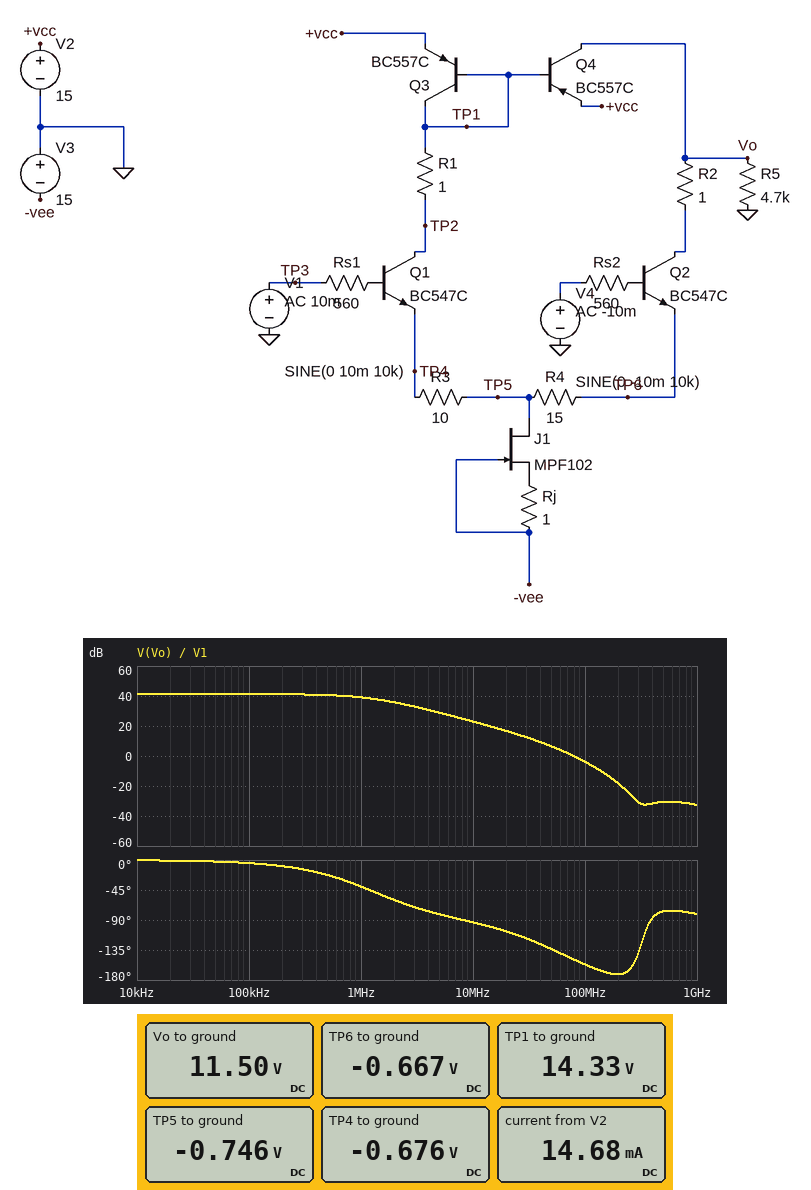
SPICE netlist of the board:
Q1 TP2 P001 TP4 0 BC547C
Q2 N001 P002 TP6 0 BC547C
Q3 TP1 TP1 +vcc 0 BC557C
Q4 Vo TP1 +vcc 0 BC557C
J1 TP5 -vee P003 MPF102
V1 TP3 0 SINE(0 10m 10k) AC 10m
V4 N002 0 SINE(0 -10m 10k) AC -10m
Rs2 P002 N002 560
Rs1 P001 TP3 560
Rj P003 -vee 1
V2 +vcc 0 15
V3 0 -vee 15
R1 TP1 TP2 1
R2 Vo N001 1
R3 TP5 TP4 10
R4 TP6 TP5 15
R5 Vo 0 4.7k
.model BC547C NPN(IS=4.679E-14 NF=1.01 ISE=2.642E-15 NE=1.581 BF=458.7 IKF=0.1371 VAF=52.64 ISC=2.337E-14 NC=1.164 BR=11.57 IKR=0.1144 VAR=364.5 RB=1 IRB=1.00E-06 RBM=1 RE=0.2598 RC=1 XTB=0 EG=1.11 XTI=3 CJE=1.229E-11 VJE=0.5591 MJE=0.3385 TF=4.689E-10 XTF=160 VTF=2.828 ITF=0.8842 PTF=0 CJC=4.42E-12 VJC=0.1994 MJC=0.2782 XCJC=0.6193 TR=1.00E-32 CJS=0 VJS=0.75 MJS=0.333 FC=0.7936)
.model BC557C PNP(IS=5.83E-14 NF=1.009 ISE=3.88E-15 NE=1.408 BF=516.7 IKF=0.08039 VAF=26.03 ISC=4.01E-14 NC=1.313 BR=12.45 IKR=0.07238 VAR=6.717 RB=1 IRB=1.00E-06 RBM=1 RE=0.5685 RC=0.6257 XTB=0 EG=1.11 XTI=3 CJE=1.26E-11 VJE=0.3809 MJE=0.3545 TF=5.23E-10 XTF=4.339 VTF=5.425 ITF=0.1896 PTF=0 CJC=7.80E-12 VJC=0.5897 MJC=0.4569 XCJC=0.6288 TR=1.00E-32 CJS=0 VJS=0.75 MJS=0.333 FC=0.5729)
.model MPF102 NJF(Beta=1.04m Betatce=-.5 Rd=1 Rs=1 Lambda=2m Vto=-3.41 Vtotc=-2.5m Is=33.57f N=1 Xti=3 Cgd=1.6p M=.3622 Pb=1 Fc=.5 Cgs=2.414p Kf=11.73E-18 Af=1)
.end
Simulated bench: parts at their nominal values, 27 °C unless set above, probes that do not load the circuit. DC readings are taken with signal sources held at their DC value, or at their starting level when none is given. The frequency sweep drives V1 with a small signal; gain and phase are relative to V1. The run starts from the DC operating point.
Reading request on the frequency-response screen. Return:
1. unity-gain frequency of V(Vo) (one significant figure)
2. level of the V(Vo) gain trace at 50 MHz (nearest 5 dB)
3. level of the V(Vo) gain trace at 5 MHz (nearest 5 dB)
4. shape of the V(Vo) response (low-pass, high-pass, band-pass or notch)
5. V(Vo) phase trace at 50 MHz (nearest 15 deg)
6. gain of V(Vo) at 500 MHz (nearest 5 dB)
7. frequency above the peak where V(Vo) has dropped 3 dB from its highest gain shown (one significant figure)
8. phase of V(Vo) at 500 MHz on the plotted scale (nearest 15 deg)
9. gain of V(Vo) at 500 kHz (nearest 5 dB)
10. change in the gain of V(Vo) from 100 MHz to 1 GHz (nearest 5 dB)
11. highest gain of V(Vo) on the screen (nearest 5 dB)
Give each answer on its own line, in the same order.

80 MHz
5 dB
30 dB
low-pass
-135 deg
-30 dB
1 MHz
-75 deg
40 dB
-30 dB
40 dB
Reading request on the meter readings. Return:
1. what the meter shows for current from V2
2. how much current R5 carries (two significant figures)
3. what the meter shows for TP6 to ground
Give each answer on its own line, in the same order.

14.68 mA
2.4 mA
-0.667 V
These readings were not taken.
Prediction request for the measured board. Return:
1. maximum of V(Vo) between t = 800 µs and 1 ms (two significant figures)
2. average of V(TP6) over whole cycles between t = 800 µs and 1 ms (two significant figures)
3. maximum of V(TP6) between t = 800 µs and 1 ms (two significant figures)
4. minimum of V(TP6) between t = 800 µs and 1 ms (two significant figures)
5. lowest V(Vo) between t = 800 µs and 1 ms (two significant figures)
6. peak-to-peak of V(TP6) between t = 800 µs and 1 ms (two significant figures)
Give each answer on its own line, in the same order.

14 V
-670 mV
-660 mV
-670 mV
9.1 V
11 mV
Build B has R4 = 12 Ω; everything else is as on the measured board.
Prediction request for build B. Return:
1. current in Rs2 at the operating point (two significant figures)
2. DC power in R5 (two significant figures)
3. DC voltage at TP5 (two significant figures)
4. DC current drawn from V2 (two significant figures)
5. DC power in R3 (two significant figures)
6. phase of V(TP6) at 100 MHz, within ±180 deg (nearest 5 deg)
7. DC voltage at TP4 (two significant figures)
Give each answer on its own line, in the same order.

11 µA
19 mW
-740 mV
14 mA
430 µW
-45 deg
-670 mV
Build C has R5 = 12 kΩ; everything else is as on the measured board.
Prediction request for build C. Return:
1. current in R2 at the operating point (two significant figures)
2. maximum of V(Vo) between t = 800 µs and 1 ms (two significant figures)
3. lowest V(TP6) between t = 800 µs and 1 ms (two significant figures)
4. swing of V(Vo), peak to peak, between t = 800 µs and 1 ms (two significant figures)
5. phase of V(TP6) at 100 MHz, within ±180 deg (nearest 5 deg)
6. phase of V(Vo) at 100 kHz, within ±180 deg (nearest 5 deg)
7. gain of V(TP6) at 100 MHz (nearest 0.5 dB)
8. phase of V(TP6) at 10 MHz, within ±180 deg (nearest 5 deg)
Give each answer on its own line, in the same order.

5.3 mA
15 V
-670 mV
2.4 V
-30 deg
0 deg
-7.0 dB
15 deg
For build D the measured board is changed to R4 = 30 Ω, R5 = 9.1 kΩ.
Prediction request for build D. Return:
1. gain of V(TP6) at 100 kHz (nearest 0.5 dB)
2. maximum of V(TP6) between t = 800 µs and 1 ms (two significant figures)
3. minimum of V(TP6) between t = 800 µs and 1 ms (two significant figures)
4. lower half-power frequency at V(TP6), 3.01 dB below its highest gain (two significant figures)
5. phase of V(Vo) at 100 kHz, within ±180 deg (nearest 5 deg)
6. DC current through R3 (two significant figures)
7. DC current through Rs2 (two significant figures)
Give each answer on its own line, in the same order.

-16.5 dB
-650 mV
-660 mV
8.7 MHz
0 deg
8.5 mA
6.6 µA
